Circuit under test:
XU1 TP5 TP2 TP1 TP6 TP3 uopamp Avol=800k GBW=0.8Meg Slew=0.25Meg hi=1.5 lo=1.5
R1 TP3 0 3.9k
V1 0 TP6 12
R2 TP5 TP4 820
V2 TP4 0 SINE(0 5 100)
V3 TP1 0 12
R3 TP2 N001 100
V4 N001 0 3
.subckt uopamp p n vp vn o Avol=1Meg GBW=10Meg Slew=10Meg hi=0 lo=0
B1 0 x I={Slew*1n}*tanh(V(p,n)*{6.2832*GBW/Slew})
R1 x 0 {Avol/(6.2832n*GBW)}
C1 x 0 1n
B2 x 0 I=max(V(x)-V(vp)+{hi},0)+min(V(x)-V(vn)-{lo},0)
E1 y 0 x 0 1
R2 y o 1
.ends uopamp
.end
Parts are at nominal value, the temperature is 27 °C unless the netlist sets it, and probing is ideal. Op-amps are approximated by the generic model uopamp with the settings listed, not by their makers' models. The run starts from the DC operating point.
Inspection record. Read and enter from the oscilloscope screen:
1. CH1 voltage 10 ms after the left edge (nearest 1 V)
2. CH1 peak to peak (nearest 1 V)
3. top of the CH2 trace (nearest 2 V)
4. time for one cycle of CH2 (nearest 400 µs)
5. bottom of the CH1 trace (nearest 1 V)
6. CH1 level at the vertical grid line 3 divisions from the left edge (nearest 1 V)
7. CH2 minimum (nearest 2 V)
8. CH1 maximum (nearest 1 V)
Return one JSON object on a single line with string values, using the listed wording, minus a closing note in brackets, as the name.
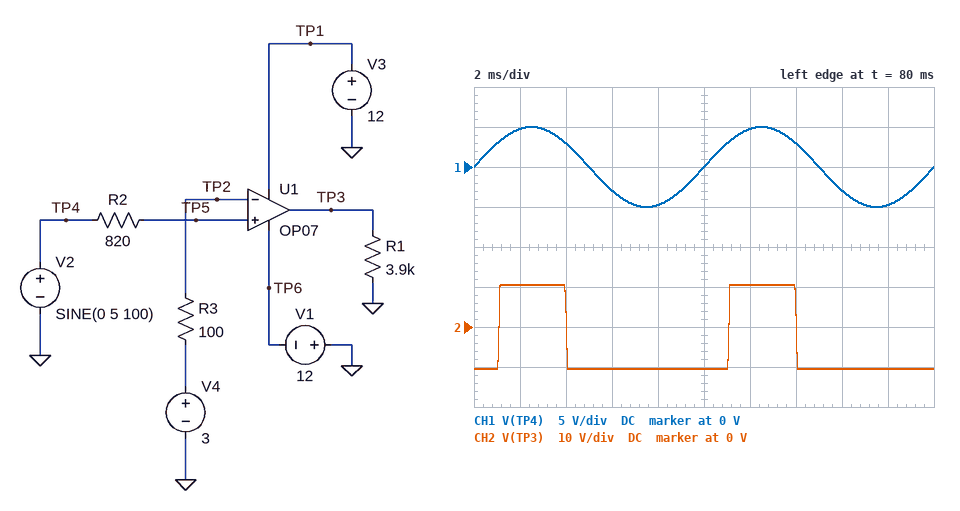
{"CH1 voltage 10 ms after the left edge": "0 V", "CH1 peak to peak": "10 V", "top of the CH2 trace": "10 V", "time for one cycle of CH2": "10.0 ms", "bottom of the CH1 trace": "-5 V", "CH1 level at the vertical grid line 3 divisions from the left edge": "-3 V", "CH2 minimum": "-10 V", "CH1 maximum": "5 V"}
